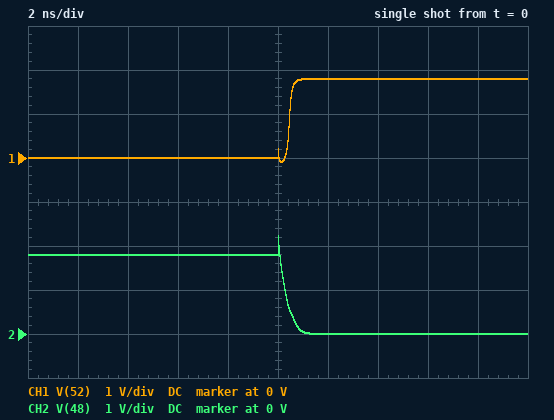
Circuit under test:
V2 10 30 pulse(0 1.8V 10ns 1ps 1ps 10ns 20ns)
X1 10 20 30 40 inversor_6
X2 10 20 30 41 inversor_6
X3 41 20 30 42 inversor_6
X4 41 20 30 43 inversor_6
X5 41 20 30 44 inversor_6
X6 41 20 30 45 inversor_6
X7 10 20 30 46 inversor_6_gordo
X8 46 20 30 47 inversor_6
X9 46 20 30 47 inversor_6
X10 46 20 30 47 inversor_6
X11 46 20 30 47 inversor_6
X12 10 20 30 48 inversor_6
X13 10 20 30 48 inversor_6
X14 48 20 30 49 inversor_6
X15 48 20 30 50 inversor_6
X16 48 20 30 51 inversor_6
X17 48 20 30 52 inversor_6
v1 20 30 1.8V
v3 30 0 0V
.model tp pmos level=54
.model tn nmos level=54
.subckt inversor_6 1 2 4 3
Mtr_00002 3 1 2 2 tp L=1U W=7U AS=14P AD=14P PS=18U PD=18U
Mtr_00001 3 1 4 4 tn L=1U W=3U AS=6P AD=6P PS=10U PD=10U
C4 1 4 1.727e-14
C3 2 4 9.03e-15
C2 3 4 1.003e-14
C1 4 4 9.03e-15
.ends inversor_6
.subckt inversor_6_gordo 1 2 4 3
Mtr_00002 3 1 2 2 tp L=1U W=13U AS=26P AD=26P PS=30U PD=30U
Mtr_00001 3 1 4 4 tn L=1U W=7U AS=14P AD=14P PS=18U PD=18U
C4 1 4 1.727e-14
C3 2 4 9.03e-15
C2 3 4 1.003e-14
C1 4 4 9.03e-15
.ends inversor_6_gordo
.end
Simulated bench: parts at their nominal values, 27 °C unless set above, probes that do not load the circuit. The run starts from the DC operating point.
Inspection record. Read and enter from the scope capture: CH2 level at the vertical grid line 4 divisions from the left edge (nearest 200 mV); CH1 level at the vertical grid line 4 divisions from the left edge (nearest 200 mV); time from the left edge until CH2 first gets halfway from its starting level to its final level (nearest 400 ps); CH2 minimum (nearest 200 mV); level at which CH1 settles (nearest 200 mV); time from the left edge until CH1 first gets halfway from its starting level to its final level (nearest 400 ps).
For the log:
1.8 V
0 V
10.4 ns
0 V
1.8 V
10.4 ns
